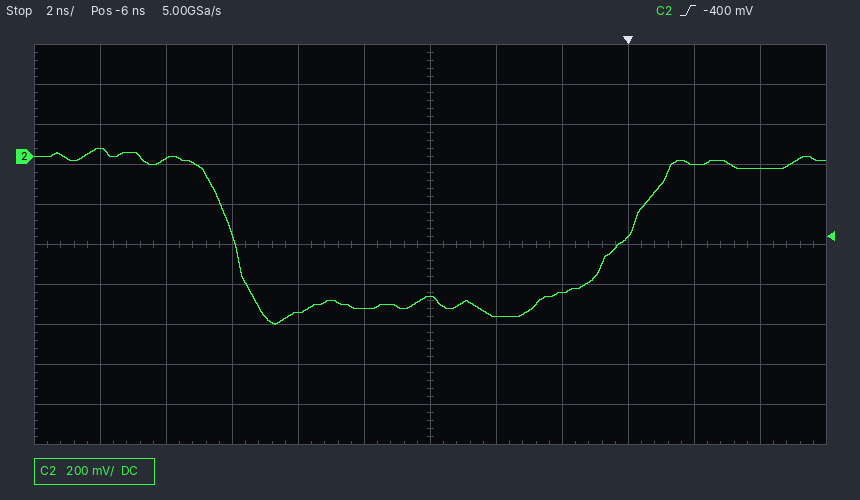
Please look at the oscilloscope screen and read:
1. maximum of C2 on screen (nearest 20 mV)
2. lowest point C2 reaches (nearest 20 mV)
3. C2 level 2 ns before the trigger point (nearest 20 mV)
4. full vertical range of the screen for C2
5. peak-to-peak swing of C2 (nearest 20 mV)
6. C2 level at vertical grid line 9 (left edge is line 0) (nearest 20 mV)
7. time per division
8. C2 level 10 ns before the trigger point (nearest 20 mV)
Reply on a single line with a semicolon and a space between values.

40 mV; -840 mV; -680 mV; 2 V; 880 mV; -400 mV; 2 ns; -780 mV
